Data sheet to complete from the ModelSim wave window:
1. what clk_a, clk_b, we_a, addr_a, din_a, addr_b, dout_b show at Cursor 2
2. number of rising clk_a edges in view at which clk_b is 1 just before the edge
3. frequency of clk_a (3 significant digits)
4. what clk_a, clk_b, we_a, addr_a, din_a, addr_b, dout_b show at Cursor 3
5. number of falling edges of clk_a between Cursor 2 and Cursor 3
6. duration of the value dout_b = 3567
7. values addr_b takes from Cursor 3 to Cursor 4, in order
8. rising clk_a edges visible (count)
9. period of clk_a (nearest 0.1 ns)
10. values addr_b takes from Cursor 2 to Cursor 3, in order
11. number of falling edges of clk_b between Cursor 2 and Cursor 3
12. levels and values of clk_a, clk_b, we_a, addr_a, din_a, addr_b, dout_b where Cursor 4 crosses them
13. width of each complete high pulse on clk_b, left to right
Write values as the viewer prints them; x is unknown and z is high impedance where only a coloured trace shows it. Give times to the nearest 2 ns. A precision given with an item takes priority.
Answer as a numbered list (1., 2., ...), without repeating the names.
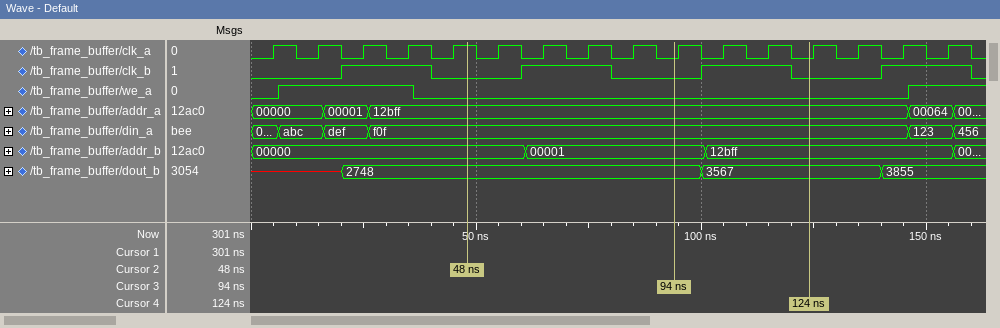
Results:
1. clk_a=1, clk_b=0, we_a=0, addr_a=12bff, din_a=f0f, addr_b=00000, dout_b=2748
2. 8
3. 100 MHz
4. clk_a=0, clk_b=0, we_a=0, addr_a=12bff, din_a=f0f, addr_b=00001, dout_b=2748
5. 5
6. 40 ns
7. 00001, 12bff
8. 16
9. 10 ns
10. 00000, 00001
11. 1
12. clk_a=0, clk_b=0, we_a=0, addr_a=12bff, din_a=f0f, addr_b=12bff, dout_b=3567
13. 20 ns, 20 ns, 20 ns, 20 ns
